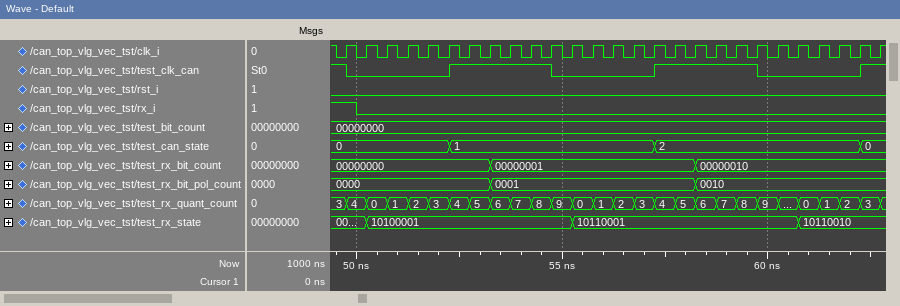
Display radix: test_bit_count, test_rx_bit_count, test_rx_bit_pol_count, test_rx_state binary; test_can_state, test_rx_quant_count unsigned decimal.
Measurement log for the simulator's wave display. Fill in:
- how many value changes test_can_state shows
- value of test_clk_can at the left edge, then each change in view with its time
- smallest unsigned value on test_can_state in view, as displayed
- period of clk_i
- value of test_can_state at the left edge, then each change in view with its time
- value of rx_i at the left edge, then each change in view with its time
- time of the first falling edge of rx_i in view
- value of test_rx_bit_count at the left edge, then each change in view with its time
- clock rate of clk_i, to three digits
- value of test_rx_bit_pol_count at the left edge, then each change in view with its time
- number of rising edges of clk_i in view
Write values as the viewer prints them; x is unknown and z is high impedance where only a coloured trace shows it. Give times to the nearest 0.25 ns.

3
1, 0 at 49.75 ns, 1 at 52.25 ns, 0 at 54.75 ns, 1 at 57.25 ns, 0 at 59.75 ns, 1 at 62.25 ns
0
0.5 ns
0, 1 at 52.25 ns, 2 at 57.25 ns, 0 at 62.25 ns
1, 0 at 50 ns
50 ns
00000000, 00000001 at 53.25 ns, 00000010 at 58.25 ns
2.00 GHz
0000, 0001 at 53.25 ns, 0010 at 58.25 ns
27
